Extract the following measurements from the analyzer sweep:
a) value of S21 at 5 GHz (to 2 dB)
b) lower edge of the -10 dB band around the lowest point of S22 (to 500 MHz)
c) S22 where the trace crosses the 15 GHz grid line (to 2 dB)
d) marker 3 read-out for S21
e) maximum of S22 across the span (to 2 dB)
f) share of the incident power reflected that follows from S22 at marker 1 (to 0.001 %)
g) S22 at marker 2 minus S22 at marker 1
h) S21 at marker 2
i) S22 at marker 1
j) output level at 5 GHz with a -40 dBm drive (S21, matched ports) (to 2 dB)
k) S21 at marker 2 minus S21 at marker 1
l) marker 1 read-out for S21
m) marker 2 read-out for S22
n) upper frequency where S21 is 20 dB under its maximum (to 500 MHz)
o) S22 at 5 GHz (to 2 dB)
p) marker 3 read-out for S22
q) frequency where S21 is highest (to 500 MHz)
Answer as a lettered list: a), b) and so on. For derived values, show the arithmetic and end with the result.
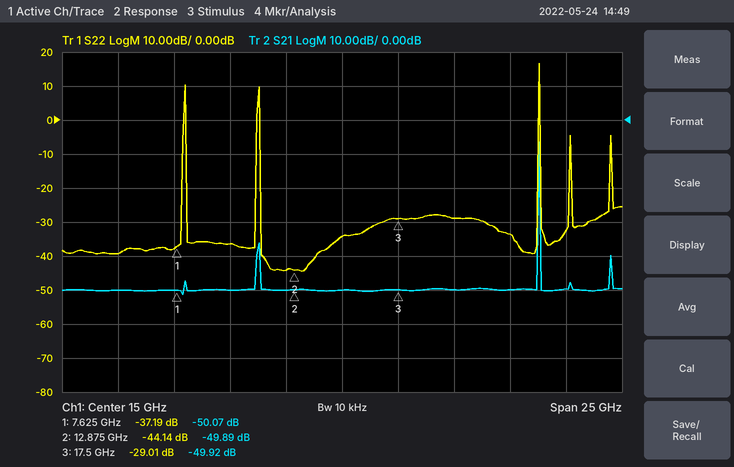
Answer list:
a) -50 dB
b) 11.5 GHz
c) -34 dB
d) -49.92 dB
e) 16 dB
f) 10^(-37.19/10) ≈ 0.019 %
g) -44.14 − (-37.19) = -6.95 dB
h) -49.89 dB
i) -37.19 dB
j) -40 dBm + (-50 dB) = -90 dBm
k) -49.89 − (-50.07) = 0.18 dB
l) -50.07 dB
m) -44.14 dB
n) 24.0 GHz
o) -40 dB
p) -29.01 dB
q) 24.0 GHz
